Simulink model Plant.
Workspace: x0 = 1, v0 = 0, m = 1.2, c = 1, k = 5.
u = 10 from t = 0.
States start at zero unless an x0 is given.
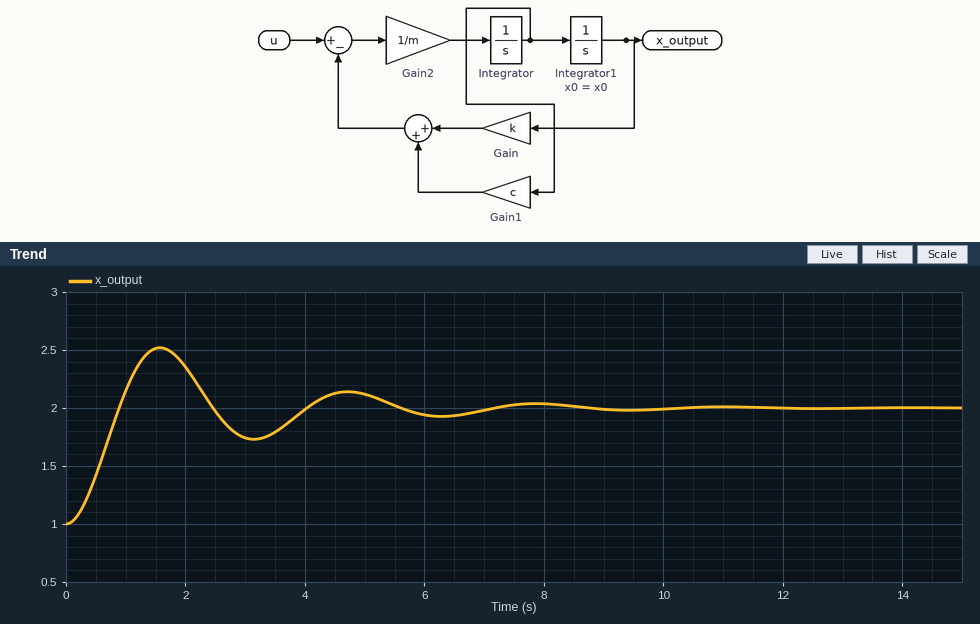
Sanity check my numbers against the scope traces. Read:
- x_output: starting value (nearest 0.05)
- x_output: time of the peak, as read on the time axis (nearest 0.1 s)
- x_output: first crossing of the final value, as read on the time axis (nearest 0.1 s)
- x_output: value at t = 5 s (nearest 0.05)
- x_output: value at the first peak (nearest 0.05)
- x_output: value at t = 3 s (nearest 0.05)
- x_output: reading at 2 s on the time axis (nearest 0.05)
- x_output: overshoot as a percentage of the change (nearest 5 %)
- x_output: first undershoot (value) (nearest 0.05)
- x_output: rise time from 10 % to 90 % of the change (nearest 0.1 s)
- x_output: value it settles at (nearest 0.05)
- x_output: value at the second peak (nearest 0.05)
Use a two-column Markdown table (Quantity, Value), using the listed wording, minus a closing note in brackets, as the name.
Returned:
| Quantity | Value |
|---|---|
| x_output: starting value | 1.00 |
| x_output: time of the peak, as read on the time axis | 1.6 s |
| x_output: first crossing of the final value, as read on the time axis | 0.9 s |
| x_output: value at t = 5 s | 2.10 |
| x_output: value at the first peak | 2.50 |
| x_output: value at t = 3 s | 1.75 |
| x_output: reading at 2 s on the time axis | 2.35 |
| x_output: overshoot as a percentage of the change | 50 % |
| x_output: first undershoot (value) | 1.75 |
| x_output: rise time from 10 % to 90 % of the change | 0.6 s |
| x_output: value it settles at | 2.00 |
| x_output: value at the second peak | 2.15 |
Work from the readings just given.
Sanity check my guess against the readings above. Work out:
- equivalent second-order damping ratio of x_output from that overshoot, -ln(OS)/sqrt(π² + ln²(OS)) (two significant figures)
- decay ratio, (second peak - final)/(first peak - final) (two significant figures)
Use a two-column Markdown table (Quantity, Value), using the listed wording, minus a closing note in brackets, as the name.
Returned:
| Quantity | Value |
|---|---|
| equivalent second-order damping ratio of x_output from that overshoot, -ln(OS)/sqrt(π² + ln²(OS)) | 0.22 |
| decay ratio, (second peak - final)/(first peak - final) | 0.30 |
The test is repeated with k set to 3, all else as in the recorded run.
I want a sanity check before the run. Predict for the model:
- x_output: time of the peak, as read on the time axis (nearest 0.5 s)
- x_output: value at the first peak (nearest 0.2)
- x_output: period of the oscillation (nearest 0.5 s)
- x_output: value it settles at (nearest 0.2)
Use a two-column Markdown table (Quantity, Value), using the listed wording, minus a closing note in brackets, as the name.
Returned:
| Quantity | Value |
|---|---|
| x_output: time of the peak, as read on the time axis | 2.0 s |
| x_output: value at the first peak | 4.4 |
| x_output: period of the oscillation | 4.0 s |
| x_output: value it settles at | 3.4 |
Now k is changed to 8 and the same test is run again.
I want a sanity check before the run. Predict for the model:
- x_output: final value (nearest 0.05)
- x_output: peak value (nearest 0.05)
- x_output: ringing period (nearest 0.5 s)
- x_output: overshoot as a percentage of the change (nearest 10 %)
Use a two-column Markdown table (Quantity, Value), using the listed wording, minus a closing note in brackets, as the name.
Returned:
| Quantity | Value |
|---|---|
| x_output: final value | 1.25 |
| x_output: peak value | 1.40 |
| x_output: ringing period | 2.5 s |
| x_output: overshoot as a percentage of the change | 60 % |
